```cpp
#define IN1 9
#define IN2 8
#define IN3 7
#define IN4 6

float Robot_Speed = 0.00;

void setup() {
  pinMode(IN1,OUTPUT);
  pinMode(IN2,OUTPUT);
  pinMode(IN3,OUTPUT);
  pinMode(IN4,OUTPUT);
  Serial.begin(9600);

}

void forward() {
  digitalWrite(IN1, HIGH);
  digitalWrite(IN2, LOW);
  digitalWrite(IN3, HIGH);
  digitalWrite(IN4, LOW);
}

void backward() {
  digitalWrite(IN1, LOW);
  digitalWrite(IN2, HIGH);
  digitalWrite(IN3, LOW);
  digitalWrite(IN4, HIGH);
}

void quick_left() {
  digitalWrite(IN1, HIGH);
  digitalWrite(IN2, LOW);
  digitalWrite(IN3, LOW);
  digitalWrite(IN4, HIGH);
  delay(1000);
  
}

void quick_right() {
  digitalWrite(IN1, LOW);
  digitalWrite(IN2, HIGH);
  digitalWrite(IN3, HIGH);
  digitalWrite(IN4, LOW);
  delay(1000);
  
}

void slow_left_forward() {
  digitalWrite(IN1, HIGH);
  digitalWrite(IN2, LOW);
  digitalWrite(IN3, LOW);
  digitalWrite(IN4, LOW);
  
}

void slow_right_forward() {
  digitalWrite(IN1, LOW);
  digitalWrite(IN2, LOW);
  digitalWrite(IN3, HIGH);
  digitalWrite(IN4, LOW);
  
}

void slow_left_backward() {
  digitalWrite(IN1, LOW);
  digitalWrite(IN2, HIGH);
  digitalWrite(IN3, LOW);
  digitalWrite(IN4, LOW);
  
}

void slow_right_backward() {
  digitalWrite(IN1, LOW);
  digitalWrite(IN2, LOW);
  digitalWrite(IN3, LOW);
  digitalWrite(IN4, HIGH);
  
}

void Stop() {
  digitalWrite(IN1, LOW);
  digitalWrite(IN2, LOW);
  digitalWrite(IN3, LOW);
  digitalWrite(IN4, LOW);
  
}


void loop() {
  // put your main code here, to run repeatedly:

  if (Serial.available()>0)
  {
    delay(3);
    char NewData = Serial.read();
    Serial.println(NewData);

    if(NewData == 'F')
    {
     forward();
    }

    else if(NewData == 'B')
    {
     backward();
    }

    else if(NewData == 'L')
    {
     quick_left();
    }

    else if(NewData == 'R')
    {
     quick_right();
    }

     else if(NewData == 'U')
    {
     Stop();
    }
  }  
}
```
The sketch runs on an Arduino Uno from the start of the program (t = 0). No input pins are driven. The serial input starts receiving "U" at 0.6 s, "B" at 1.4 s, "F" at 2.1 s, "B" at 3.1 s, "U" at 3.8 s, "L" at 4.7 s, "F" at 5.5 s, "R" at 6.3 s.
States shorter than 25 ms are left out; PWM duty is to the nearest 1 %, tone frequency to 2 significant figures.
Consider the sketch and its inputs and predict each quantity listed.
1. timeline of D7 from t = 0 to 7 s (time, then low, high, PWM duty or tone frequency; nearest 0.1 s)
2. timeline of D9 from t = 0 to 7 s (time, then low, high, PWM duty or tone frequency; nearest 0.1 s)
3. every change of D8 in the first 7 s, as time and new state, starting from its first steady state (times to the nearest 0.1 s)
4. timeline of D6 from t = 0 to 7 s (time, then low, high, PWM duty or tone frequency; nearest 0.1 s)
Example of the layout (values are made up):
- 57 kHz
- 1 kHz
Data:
- 0 s low; 2.1 s high; 3.1 s low; 5.7 s high
- 0 s low; 2.1 s high; 3.1 s low; 4.7 s high; 6.3 s low
- 0 s low; 1.4 s high; 2.1 s low; 3.1 s high; 3.8 s low; 6.3 s high
- 0 s low; 1.4 s high; 2.1 s low; 3.1 s high; 3.8 s low; 4.7 s high; 5.7 s low
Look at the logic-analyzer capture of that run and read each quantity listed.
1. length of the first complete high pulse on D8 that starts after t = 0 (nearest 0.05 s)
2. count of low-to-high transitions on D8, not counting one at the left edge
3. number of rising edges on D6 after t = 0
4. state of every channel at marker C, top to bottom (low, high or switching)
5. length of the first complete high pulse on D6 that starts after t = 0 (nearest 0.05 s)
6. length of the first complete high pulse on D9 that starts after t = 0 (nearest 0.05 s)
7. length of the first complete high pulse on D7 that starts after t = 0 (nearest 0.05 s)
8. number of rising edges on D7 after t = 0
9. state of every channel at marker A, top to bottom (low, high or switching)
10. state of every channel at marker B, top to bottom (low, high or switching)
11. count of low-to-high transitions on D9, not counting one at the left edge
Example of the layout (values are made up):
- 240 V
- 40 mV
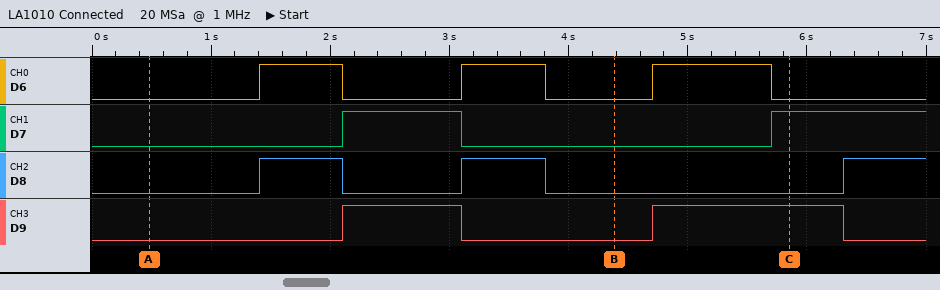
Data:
- 0.70 s
- 3
- 3
- D6 low, D7 high, D8 low, D9 high
- 0.70 s
- 1.00 s
- 1.00 s
- 2
- D6 low, D7 low, D8 low, D9 low
- D6 low, D7 low, D8 low, D9 low
- 2
